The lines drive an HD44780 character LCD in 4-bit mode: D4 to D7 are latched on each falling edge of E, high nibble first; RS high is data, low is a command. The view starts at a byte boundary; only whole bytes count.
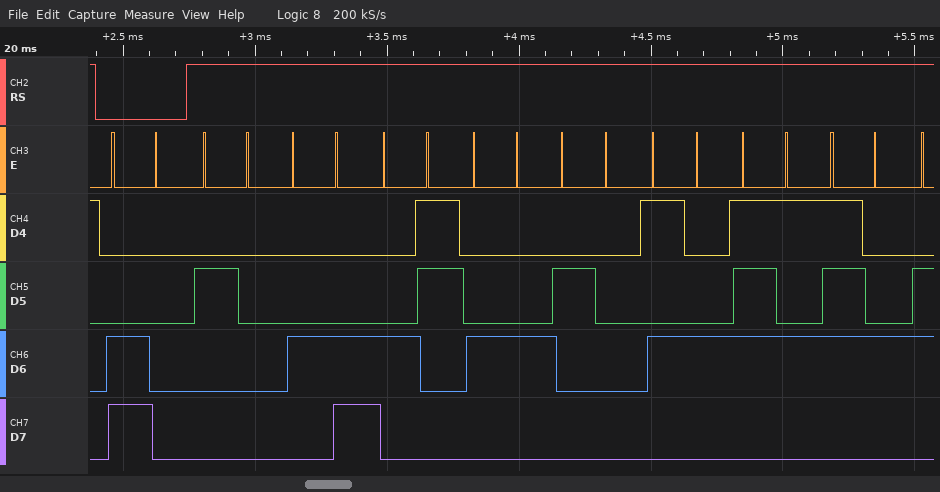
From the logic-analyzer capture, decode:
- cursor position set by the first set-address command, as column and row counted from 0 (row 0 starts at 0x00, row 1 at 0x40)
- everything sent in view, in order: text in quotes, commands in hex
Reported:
column 0, row 1
0xC0 " LCD Tut"
